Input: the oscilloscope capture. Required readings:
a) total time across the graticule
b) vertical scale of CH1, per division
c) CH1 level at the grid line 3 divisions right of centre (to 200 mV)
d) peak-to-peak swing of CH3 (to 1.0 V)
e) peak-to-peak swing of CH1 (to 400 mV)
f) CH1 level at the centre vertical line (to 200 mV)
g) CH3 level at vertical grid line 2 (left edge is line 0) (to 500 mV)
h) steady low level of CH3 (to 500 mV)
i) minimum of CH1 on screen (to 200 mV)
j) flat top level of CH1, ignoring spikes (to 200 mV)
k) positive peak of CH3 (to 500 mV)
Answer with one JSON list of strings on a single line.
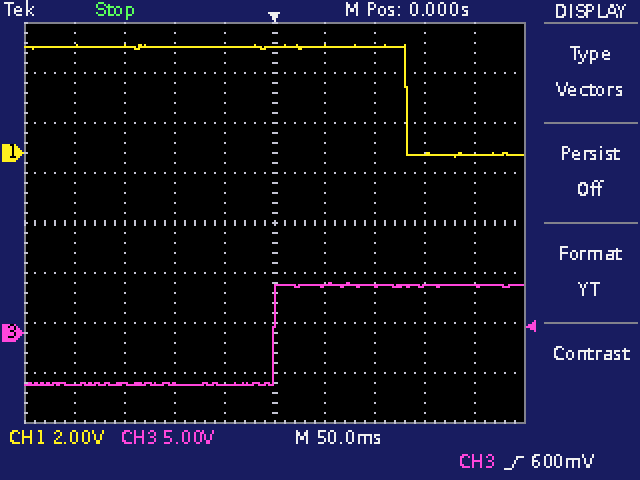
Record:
["500 ms", "2 V", "0.0 V", "10.0 V", "4.4 V", "4.2 V", "-5.0 V", "-5.0 V", "-200 mV", "4.2 V", "5.0 V"]
